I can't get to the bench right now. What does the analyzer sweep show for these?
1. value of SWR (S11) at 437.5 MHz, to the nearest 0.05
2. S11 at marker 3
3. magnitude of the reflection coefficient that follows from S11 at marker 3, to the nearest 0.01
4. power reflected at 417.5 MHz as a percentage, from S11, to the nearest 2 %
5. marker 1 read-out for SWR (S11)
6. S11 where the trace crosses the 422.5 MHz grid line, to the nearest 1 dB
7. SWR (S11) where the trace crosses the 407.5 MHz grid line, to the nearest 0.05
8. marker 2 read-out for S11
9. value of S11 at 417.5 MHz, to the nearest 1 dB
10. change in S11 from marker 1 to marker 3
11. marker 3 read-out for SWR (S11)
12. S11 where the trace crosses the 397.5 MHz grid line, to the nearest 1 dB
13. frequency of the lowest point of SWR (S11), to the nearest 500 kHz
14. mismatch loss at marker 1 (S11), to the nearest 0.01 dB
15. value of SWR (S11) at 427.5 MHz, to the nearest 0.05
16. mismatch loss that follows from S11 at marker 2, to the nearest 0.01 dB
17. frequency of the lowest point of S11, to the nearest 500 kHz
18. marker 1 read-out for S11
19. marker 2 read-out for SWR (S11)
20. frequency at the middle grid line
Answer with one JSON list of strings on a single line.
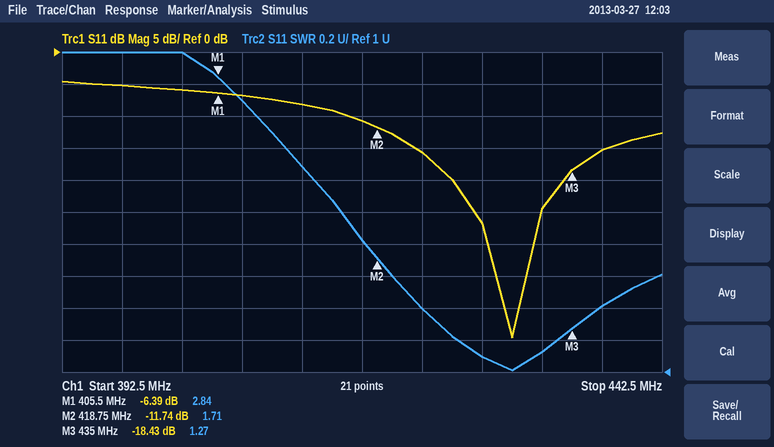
["1.40", "-18.43 dB", "0.12", "8 %", "2.84", "-16 dB", "2.70", "-11.74 dB", "-11 dB", "-12.04 dB", "1.27", "-5 dB", "430.0 MHz", "1.13 dB", "1.10", "0.30 dB", "430.0 MHz", "-6.39 dB", "1.71", "417.5 MHz"]
